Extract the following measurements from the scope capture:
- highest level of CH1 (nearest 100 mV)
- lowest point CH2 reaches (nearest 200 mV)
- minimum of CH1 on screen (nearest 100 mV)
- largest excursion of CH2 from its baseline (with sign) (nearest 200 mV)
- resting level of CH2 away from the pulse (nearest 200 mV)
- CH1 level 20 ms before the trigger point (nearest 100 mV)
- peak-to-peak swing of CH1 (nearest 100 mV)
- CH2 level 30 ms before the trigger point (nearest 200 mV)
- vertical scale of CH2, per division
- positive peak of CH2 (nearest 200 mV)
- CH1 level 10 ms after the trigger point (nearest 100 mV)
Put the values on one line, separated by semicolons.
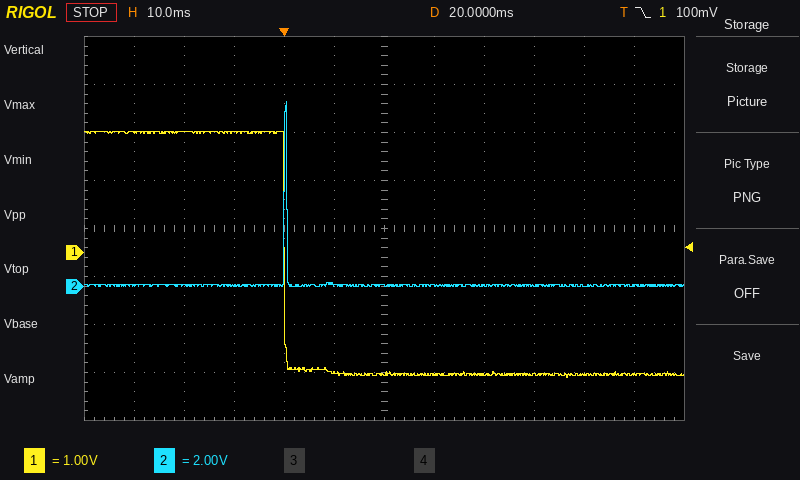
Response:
2.5 V; 0.0 V; -2.6 V; +7.6 V; 0.0 V; 2.5 V; 5.1 V; 0.0 V; 2 V; 7.6 V; -2.5 V
